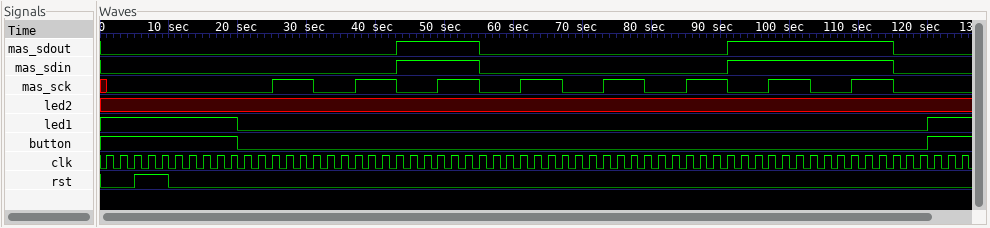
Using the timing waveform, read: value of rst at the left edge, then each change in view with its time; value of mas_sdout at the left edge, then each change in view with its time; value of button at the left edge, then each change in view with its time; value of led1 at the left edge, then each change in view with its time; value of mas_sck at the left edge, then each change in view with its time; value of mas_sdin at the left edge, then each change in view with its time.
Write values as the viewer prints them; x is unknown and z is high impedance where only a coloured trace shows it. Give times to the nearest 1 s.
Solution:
0, 1 at 5 s, 0 at 10 s
0, 1 at 43 s, 0 at 55 s, 1 at 91 s, 0 at 115 s
1, 0 at 20 s, 1 at 120 s
1, 0 at 20 s, 1 at 120 s
x, 0 at 1 s, 1 at 25 s, 0 at 31 s, 1 at 37 s, 0 at 43 s, 1 at 49 s, 0 at 55 s, 1 at 61 s, 0 at 67 s, 1 at 73 s, 0 at 79 s, 1 at 85 s, 0 at 91 s, 1 at 97 s, 0 at 103 s, 1 at 109 s, 0 at 115 s
0, 1 at 43 s, 0 at 55 s, 1 at 91 s, 0 at 115 s
